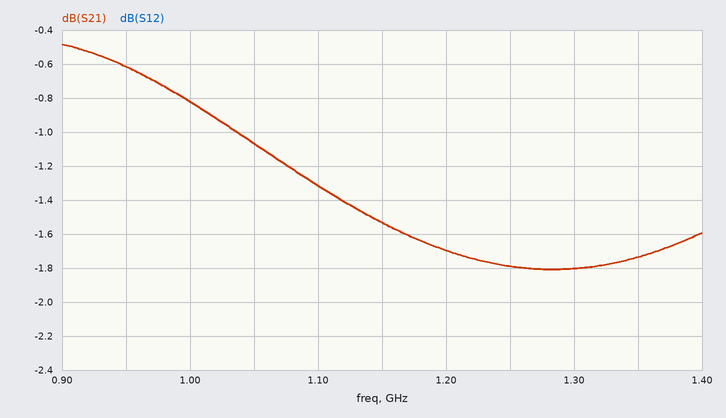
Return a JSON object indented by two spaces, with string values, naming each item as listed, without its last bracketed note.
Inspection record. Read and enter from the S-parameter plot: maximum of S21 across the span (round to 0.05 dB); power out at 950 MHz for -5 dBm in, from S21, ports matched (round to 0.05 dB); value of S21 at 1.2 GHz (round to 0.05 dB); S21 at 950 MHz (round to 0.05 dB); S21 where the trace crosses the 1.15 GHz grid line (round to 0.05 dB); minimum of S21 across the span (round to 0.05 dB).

{
  "maximum of S21 across the span": "-0.50 dB",
  "power out at 950 MHz for -5 dBm in, from S21, ports matched": "-5.60 dBm",
  "value of S21 at 1.2 GHz": "-1.70 dB",
  "S21 at 950 MHz": "-0.60 dB",
  "S21 where the trace crosses the 1.15 GHz grid line": "-1.55 dB",
  "minimum of S21 across the span": "-1.80 dB"
}
